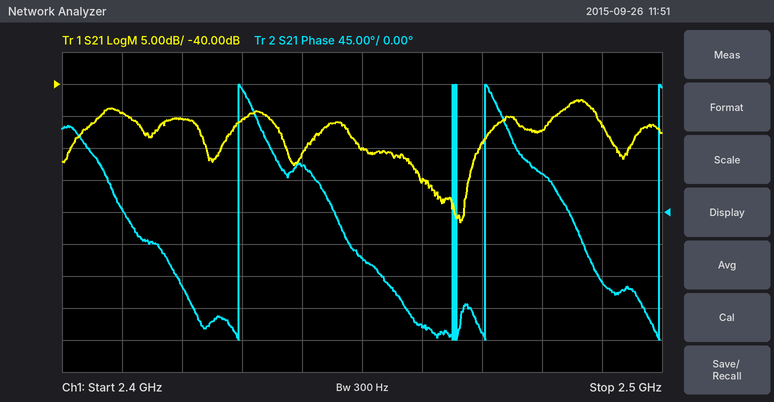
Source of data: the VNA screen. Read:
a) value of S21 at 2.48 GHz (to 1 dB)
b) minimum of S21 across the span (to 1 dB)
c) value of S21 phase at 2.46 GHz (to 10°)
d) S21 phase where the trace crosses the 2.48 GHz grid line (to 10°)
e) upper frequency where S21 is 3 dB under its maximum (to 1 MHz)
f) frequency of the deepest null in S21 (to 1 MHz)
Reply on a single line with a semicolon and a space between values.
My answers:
-47 dB; -62 dB; -160°; 50°; 2.489 GHz; 2.466 GHz
